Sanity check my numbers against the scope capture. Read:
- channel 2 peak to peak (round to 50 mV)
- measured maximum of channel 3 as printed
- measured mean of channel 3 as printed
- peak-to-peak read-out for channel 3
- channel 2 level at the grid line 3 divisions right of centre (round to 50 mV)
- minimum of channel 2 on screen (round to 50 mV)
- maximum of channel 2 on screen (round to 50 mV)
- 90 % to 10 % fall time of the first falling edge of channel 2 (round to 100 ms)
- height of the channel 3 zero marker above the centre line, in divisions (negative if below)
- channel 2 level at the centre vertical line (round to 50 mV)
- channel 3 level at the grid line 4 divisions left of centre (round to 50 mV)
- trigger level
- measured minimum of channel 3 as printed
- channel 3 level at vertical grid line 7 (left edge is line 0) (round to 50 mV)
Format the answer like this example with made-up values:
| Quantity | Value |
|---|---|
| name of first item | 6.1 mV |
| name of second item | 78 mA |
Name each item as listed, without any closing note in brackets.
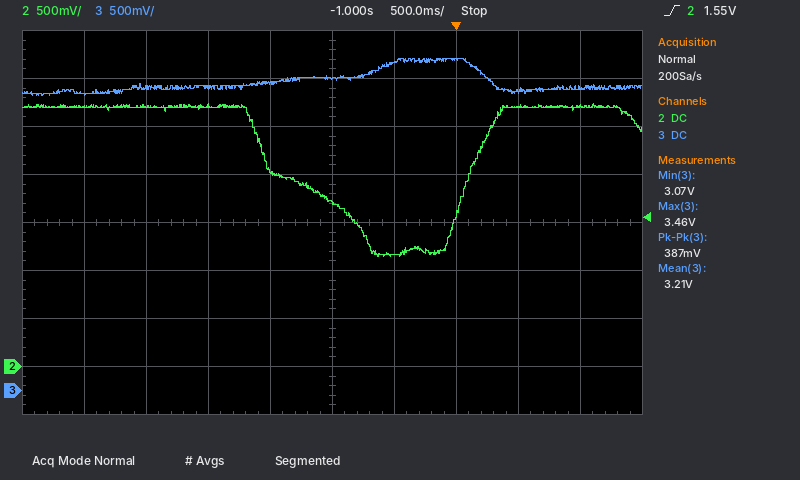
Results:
| Quantity | Value |
|---|---|
| channel 2 peak to peak | 1.60 V |
| measured maximum of channel 3 as printed | 3.46 V |
| measured mean of channel 3 as printed | 3.21 V |
| peak-to-peak read-out for channel 3 | 387 mV |
| channel 2 level at the grid line 3 divisions right of centre | 2.70 V |
| minimum of channel 2 on screen | 1.15 V |
| maximum of channel 2 on screen | 2.75 V |
| 90 % to 10 % fall time of the first falling edge of channel 2 | 900 ms |
| height of the channel 3 zero marker above the centre line, in divisions | -3.5 div |
| channel 2 level at the centre vertical line | 1.70 V |
| channel 3 level at the grid line 4 divisions left of centre | 3.10 V |
| trigger level | 1.55 V |
| measured minimum of channel 3 as printed | 3.07 V |
| channel 3 level at vertical grid line 7 (left edge is line 0) | 3.45 V |
